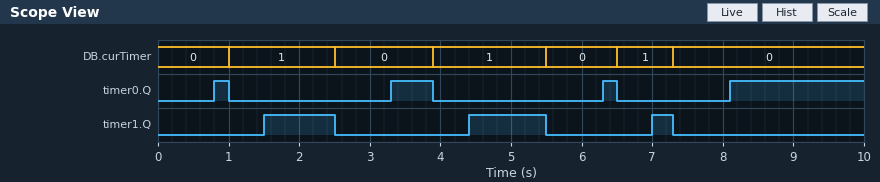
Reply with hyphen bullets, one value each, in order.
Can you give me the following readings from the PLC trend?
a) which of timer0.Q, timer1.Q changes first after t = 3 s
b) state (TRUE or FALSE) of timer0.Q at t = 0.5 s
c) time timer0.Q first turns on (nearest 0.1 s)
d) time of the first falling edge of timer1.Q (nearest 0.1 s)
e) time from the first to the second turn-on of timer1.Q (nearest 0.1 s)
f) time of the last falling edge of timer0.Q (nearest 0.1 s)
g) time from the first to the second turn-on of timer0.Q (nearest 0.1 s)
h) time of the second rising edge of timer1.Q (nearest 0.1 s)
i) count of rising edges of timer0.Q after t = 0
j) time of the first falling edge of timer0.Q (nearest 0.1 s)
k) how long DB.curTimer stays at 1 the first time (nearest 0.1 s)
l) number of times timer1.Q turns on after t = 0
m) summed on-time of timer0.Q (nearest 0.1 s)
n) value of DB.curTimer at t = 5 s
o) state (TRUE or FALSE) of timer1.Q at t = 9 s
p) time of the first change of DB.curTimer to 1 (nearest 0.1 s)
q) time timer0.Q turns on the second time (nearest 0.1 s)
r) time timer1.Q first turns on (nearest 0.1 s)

- timer0.Q
- FALSE
- 0.8 s
- 2.5 s
- 2.9 s
- 6.5 s
- 2.5 s
- 4.4 s
- 4
- 1.0 s
- 1.5 s
- 3
- 2.9 s
- 1
- FALSE
- 1.0 s
- 3.3 s
- 1.5 s
